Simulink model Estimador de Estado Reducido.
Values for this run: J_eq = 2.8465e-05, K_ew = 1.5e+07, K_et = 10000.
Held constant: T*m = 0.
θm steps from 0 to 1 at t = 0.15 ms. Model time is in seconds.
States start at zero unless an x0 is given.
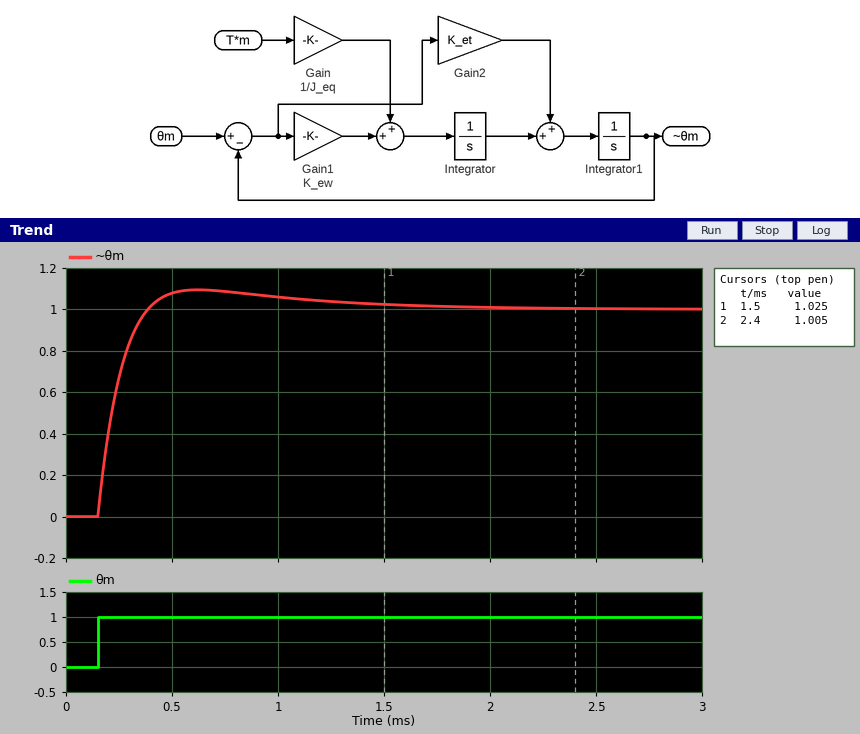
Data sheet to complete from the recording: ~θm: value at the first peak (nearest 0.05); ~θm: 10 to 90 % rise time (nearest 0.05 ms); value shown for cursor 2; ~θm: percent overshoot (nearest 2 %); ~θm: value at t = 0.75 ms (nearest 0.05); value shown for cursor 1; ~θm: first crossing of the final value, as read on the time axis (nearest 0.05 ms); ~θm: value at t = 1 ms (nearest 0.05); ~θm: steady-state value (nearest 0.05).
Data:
1.10
0.15 ms
1.005
10 %
1.10
1.025
0.40 ms
1.05
1.00
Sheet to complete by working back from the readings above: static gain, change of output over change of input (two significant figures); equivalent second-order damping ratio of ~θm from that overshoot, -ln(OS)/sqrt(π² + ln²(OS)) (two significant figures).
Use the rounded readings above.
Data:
1.0
0.59
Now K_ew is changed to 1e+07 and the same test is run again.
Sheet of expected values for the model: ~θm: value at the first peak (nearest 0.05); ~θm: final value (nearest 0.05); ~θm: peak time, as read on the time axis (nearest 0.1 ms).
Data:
1.05
1.00
0.7 ms
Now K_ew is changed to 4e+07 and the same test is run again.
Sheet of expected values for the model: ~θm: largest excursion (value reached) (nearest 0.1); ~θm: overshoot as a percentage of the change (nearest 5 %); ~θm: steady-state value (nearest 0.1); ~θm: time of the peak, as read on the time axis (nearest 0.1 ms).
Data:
1.2
20 %
1.0
0.5 ms
